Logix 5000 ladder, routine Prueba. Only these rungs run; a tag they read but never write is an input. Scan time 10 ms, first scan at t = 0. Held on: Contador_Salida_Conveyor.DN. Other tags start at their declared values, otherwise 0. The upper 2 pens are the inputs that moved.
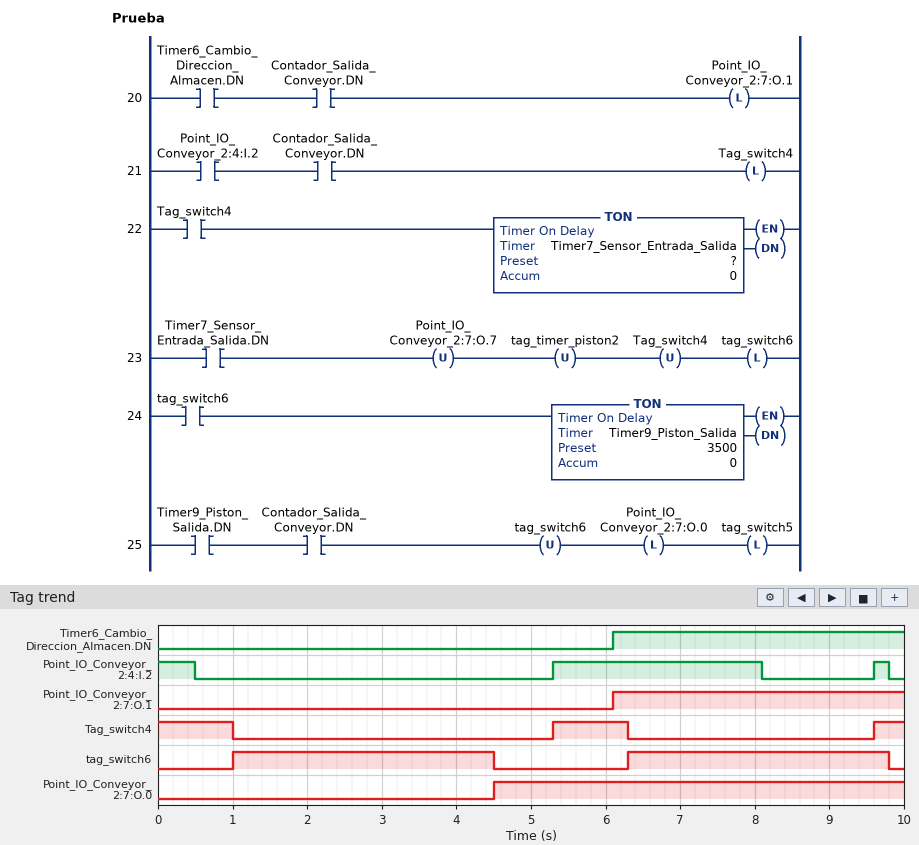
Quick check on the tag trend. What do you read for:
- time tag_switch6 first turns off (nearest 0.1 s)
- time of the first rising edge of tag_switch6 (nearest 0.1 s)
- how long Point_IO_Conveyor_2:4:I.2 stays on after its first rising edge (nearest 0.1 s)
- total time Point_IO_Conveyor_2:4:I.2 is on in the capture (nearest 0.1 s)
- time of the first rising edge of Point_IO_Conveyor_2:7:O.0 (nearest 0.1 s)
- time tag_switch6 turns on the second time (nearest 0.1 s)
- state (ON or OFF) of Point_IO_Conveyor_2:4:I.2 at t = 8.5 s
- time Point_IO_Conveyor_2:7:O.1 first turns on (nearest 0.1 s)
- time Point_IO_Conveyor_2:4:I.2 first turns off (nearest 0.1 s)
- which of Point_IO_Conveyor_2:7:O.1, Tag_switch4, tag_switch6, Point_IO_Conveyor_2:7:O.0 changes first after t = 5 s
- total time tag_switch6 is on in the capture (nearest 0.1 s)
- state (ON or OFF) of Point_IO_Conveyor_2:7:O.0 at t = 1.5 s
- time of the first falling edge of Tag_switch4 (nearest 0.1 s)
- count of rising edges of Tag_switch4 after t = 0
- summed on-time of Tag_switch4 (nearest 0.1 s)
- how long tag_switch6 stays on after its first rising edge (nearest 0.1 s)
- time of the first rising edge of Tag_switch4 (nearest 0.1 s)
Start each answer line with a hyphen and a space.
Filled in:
- 4.5 s
- 1.0 s
- 2.8 s
- 3.5 s
- 4.5 s
- 6.3 s
- OFF
- 6.1 s
- 0.5 s
- Tag_switch4
- 7.0 s
- OFF
- 1.0 s
- 2
- 2.4 s
- 3.5 s
- 5.3 s
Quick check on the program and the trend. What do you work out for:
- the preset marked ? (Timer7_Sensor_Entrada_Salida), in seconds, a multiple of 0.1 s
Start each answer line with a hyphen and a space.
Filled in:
- 1.0 s
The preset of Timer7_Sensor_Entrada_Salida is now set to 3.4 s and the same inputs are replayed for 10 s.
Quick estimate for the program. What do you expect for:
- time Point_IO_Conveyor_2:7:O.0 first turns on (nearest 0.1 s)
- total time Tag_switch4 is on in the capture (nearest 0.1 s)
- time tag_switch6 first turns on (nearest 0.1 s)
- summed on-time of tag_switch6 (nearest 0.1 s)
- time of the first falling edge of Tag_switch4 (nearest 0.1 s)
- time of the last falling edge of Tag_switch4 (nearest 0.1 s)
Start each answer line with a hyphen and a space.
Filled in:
- 6.9 s
- 7.2 s
- 3.4 s
- 4.8 s
- 3.4 s
- 8.7 s
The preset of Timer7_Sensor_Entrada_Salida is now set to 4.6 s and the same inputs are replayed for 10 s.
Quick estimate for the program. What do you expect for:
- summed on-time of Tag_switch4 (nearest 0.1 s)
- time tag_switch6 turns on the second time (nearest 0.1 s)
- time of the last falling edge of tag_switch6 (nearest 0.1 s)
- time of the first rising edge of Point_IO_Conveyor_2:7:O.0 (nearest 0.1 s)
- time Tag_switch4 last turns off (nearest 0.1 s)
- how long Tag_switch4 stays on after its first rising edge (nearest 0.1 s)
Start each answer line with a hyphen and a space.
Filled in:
- 9.2 s
- 9.9 s
- 8.1 s
- 8.1 s
- 9.9 s
- 4.6 s
